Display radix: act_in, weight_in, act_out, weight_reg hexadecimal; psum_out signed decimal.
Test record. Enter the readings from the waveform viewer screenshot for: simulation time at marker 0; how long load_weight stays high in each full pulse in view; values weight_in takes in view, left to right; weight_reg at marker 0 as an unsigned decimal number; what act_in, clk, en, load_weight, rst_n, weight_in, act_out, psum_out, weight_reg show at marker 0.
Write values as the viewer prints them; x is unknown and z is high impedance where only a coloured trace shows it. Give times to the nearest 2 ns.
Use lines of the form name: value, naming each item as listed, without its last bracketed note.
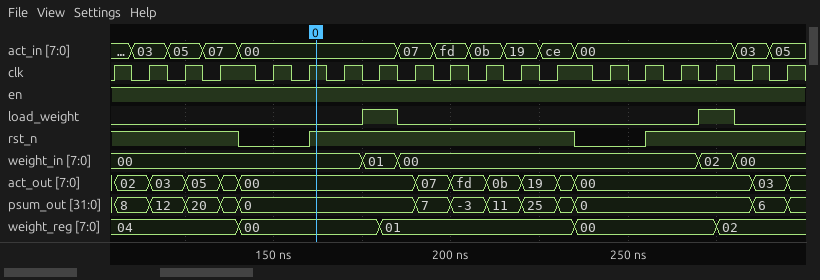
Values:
simulation time at marker 0: 162 ns
how long load_weight stays high in each full pulse in view: 10 ns, 10 ns
values weight_in takes in view, left to right: 00, 01, 00, 02, 00
weight_reg at marker 0 as an unsigned decimal number: 0
what act_in, clk, en, load_weight, rst_n, weight_in, act_out, psum_out, weight_reg show at marker 0: act_in=00, clk=1, en=1, load_weight=0, rst_n=1, weight_in=00, act_out=00, psum_out=0, weight_reg=00
